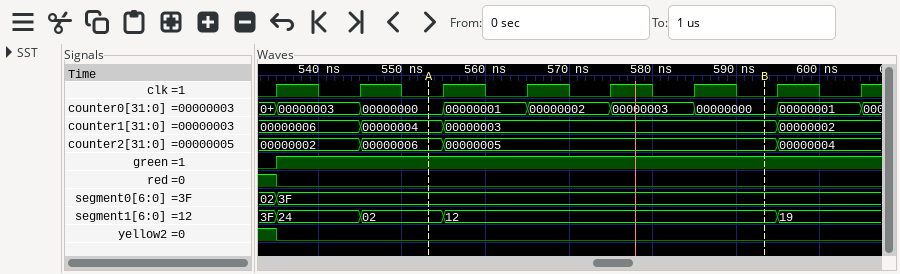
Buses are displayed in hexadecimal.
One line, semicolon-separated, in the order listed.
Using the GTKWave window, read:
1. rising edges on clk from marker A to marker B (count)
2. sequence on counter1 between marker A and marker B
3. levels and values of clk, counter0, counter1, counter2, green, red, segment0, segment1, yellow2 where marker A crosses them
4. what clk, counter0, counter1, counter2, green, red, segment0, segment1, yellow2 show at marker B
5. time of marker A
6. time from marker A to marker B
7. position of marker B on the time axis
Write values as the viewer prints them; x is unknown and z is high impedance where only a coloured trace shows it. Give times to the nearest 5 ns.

4; 00000004, 00000003; clk=0, counter0=00000000, counter1=00000004, counter2=00000006, green=1, red=0, segment0=3F, segment1=02, yellow2=0; clk=0, counter0=00000000, counter1=00000003, counter2=00000005, green=1, red=0, segment0=3F, segment1=12, yellow2=0; 555 ns; 40 ns; 595 ns
